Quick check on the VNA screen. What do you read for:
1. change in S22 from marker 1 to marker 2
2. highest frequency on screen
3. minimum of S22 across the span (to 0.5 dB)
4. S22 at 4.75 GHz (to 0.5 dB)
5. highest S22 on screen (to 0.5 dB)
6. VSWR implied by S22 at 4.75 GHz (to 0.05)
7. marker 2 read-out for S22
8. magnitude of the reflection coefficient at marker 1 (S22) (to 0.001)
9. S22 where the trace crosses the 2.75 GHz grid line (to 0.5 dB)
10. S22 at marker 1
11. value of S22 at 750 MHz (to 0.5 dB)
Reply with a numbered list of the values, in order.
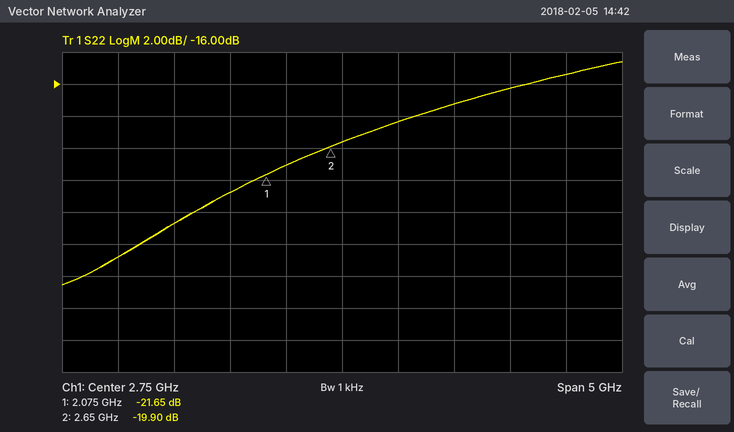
1. 1.75 dB
2. 5.25 GHz
3. -28.5 dB
4. -15.5 dB
5. -14.5 dB
6. 1.40
7. -19.90 dB
8. 0.083
9. -19.5 dB
10. -21.65 dB
11. -27.0 dB
